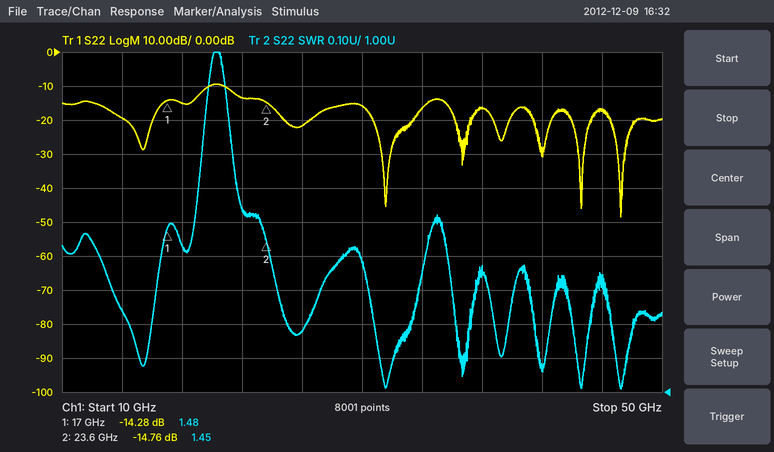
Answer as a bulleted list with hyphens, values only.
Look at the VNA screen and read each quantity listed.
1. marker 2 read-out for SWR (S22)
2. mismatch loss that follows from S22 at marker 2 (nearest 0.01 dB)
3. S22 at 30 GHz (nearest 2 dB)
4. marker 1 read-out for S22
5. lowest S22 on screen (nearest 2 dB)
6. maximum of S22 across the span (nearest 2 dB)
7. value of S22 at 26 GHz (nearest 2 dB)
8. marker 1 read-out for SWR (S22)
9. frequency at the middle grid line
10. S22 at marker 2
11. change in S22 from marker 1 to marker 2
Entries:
- 1.45
- 0.15 dB
- -16 dB
- -14.28 dB
- -48 dB
- -10 dB
- -22 dB
- 1.48
- 30 GHz
- -14.76 dB
- -0.48 dB
